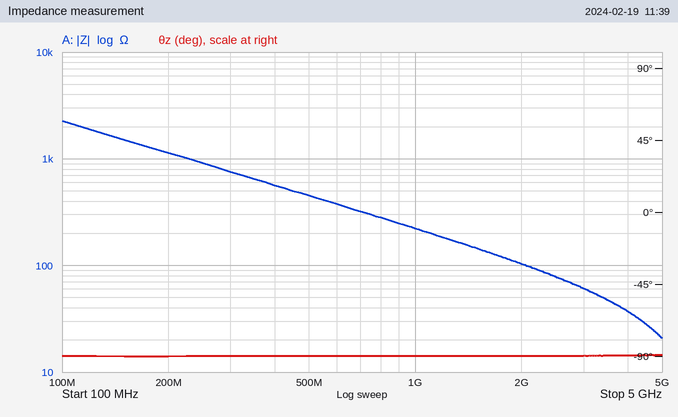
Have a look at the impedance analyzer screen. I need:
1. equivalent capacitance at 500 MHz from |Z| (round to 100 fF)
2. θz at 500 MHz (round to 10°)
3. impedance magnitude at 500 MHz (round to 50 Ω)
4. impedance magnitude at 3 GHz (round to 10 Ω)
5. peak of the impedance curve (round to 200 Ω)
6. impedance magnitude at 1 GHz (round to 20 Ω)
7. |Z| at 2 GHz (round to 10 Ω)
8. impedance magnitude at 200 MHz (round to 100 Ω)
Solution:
700 fF
-90°
450 Ω
60 Ω
2.2 kΩ
220 Ω
100 Ω
1.1 kΩ
